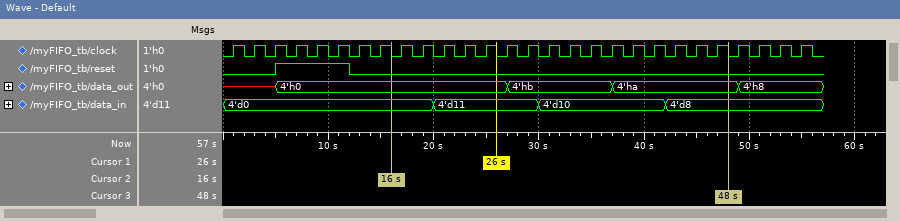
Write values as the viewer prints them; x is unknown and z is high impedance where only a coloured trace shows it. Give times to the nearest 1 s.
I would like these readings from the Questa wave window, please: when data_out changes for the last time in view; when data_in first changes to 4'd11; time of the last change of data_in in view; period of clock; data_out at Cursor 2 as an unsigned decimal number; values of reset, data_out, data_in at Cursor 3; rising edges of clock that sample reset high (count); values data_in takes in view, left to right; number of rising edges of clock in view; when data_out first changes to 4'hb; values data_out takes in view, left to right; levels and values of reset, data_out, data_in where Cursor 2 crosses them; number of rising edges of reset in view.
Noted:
49 s
20 s
42 s
2 s
0
reset=0, data_out=4'ha, data_in=4'd8
3
4'd0, 4'd11, 4'd10, 4'd8
28
27 s
x, 4'h0, 4'hb, 4'ha, 4'h8
reset=0, data_out=4'h0, data_in=4'd0
1
